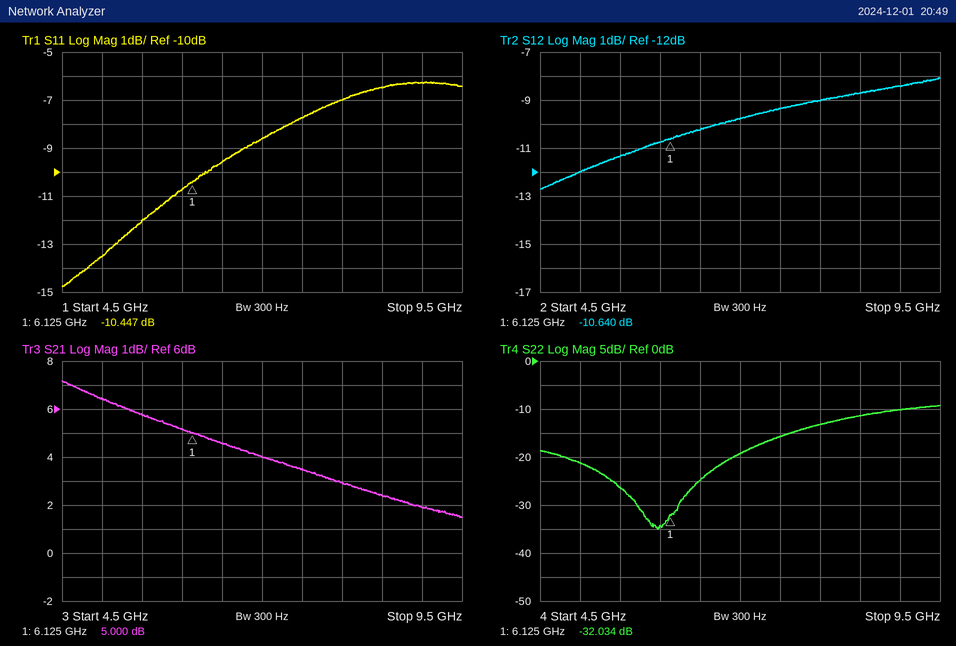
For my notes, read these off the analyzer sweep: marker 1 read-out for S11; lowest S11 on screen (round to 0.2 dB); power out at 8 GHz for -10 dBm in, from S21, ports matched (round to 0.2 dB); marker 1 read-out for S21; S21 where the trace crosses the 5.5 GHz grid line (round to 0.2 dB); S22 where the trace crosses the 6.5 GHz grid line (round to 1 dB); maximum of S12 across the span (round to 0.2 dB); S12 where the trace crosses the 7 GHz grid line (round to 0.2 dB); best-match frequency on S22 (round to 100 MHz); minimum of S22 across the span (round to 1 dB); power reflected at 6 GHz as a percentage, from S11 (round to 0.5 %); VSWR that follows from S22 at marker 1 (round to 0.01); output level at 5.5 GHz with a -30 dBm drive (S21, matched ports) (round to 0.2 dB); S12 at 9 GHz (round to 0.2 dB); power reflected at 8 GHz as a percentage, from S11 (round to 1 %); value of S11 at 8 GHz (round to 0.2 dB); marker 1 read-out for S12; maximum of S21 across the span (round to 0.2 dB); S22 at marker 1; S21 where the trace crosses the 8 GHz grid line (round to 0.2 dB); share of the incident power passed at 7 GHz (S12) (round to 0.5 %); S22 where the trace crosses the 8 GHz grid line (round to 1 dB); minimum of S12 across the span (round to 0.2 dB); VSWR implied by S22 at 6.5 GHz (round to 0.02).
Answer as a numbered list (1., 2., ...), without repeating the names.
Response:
1. -10.447 dB
2. -14.8 dB
3. -7.0 dBm
4. 5.000 dB
5. 5.8 dB
6. -25 dB
7. -8.0 dB
8. -9.8 dB
9. 6.0 GHz
10. -35 dB
11. 8.5 %
12. 1.05
13. -24.2 dBm
14. -8.4 dB
15. 20 %
16. -7.0 dB
17. -10.640 dB
18. 7.2 dB
19. -32.034 dB
20. 3.0 dB
21. 10.5 %
22. -13 dB
23. -12.8 dB
24. 1.12
